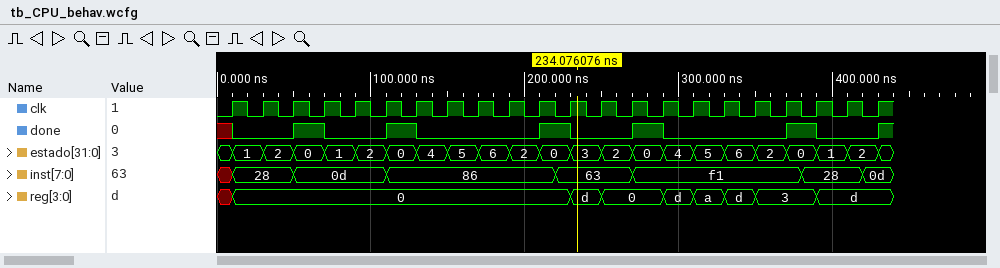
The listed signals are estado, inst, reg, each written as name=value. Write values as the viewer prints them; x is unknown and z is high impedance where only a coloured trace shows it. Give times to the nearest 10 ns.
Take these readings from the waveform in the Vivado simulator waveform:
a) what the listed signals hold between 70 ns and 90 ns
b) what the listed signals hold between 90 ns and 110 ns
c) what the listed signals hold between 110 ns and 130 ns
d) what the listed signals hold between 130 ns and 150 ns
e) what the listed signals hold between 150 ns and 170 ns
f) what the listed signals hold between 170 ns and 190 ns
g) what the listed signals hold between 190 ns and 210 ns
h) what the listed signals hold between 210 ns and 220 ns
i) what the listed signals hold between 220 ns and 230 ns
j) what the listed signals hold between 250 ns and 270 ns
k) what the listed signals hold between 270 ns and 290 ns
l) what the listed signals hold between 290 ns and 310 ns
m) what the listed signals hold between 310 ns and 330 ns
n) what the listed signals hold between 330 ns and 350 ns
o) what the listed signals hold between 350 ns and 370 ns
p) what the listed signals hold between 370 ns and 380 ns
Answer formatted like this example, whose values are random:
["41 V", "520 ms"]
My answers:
["estado=1, inst=0d, reg=0", "estado=2, inst=0d, reg=0", "estado=0, inst=86, reg=0", "estado=4, inst=86, reg=0", "estado=5, inst=86, reg=0", "estado=6, inst=86, reg=0", "estado=2, inst=86, reg=0", "estado=0, inst=86, reg=0", "estado=0, inst=63, reg=0", "estado=2, inst=63, reg=0", "estado=0, inst=f1, reg=0", "estado=4, inst=f1, reg=d", "estado=5, inst=f1, reg=a", "estado=6, inst=f1, reg=d", "estado=2, inst=f1, reg=3", "estado=0, inst=f1, reg=3"]
